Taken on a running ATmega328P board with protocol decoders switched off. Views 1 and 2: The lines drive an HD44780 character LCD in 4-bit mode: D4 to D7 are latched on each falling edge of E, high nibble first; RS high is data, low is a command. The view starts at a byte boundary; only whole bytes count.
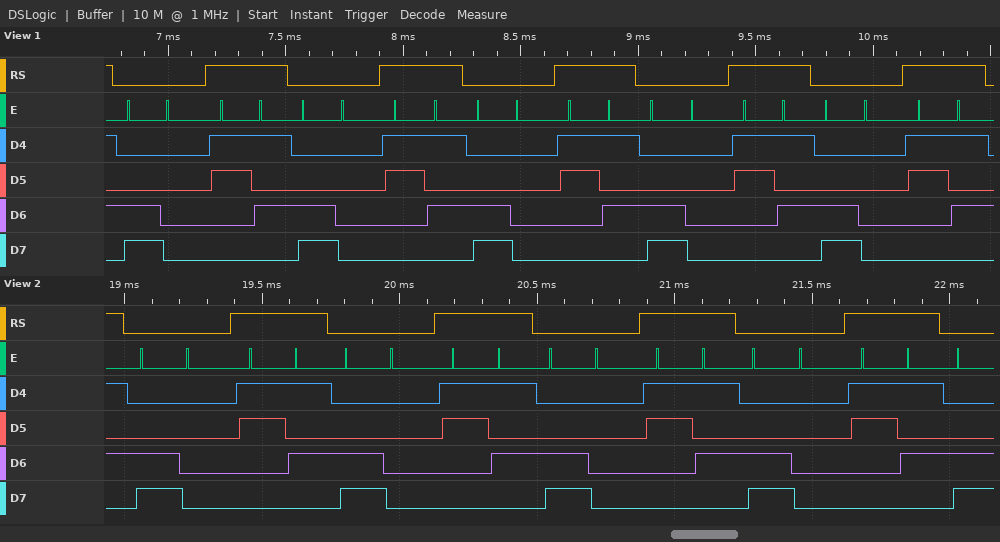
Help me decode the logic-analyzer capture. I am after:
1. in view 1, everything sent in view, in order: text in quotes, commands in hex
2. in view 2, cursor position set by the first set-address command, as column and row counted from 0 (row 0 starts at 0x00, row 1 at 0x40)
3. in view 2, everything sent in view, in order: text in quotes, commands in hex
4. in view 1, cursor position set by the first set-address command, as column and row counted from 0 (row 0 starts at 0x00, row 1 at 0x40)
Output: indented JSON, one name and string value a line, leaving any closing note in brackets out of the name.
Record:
{
  "in view 1, everything sent in view, in order: text in quotes, commands in hex": "0xC0 \"5\" 0xC0 \"5\" 0xC0 \"5\" 0xC0 \"5\" 0xC0 \"5\"",
  "in view 2, cursor position set by the first set-address command, as column and row counted from 0": "column 0, row 1",
  "in view 2, everything sent in view, in order: text in quotes, commands in hex": "0xC0 \"5\" 0xC0 \"5\" 0xC0 \"5\" 0xC0 \"5\"",
  "in view 1, cursor position set by the first set-address command, as column and row counted from 0": "column 0, row 1"
}
